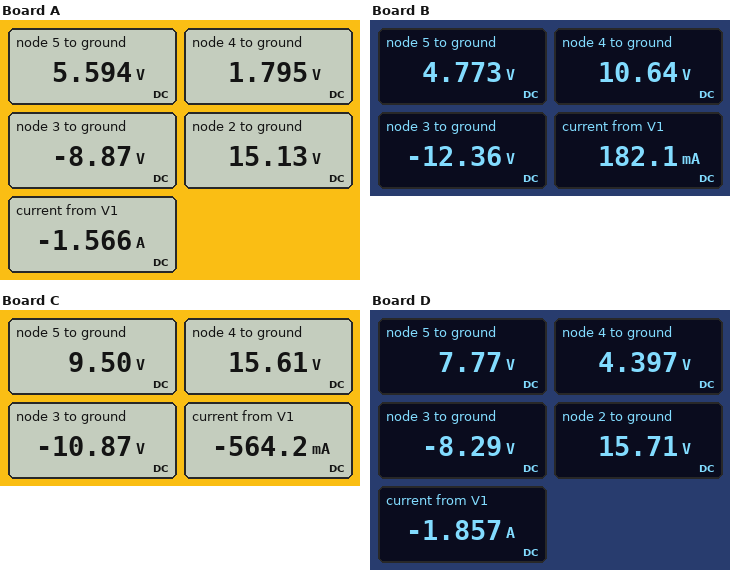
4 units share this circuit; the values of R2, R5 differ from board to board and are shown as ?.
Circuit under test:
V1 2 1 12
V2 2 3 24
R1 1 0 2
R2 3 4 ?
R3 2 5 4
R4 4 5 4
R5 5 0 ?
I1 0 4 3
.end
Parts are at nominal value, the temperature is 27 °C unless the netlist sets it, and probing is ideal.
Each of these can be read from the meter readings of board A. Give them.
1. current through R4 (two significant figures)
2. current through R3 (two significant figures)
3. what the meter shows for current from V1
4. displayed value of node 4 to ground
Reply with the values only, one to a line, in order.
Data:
950 mA
2.4 A
-1.566 A
1.795 V
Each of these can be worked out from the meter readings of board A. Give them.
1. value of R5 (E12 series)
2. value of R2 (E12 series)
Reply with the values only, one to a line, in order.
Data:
3.9 Ω
2.7 Ω
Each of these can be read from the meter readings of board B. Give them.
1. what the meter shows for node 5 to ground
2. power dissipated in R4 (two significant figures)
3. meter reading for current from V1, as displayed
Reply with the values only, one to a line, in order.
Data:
4.773 V
8.6 W
182.1 mA
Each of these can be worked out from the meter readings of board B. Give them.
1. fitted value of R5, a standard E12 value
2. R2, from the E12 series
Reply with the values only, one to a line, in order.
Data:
1.5 Ω
15 Ω
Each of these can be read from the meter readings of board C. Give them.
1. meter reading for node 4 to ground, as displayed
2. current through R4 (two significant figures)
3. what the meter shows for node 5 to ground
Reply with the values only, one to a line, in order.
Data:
15.61 V
1.5 A
9.50 V
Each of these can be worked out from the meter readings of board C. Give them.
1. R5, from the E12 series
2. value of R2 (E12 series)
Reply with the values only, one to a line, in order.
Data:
3.9 Ω
18 Ω
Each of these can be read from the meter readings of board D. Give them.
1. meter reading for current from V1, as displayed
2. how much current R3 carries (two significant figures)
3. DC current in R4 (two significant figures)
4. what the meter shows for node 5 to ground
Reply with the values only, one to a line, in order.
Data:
-1.857 A
2.0 A
840 mA
7.77 V
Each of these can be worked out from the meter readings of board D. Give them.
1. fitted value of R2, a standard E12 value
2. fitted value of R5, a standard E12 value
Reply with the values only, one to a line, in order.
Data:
3.3 Ω
6.8 Ω
